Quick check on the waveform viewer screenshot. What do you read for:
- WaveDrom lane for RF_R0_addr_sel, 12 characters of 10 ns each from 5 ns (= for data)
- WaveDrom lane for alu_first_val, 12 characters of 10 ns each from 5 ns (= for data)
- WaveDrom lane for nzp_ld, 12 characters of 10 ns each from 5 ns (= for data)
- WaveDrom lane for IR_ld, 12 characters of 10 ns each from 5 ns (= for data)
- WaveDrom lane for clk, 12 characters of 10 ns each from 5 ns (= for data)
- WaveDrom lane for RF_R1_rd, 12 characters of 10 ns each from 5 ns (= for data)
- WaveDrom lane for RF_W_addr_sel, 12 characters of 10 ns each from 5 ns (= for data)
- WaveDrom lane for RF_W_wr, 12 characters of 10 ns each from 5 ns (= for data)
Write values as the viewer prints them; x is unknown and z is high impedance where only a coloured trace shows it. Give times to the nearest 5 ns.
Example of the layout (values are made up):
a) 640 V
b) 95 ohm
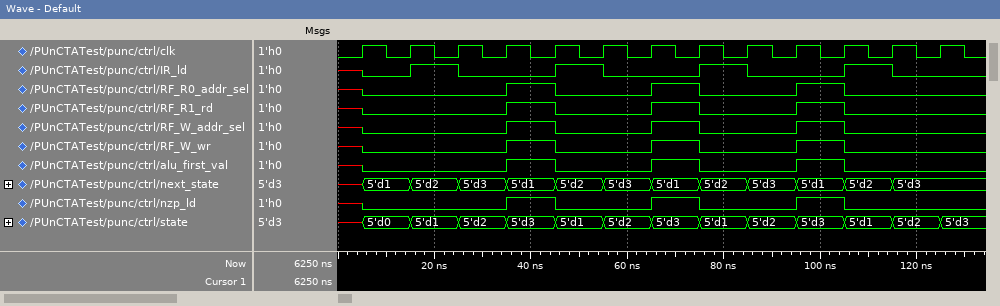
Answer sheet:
a) {name: 'RF_R0_addr_sel', wave: '0..10.10.10.'}
b) {name: 'alu_first_val', wave: '0..10.10.10.'}
c) {name: 'nzp_ld', wave: '0..10.10.10.'}
d) {name: 'IR_ld', wave: '010.10.10.10'}
e) {name: 'clk', wave: 'p...........'}
f) {name: 'RF_R1_rd', wave: '0..10.10.10.'}
g) {name: 'RF_W_addr_sel', wave: '0..10.10.10.'}
h) {name: 'RF_W_wr', wave: '0..10.10.10.'}
